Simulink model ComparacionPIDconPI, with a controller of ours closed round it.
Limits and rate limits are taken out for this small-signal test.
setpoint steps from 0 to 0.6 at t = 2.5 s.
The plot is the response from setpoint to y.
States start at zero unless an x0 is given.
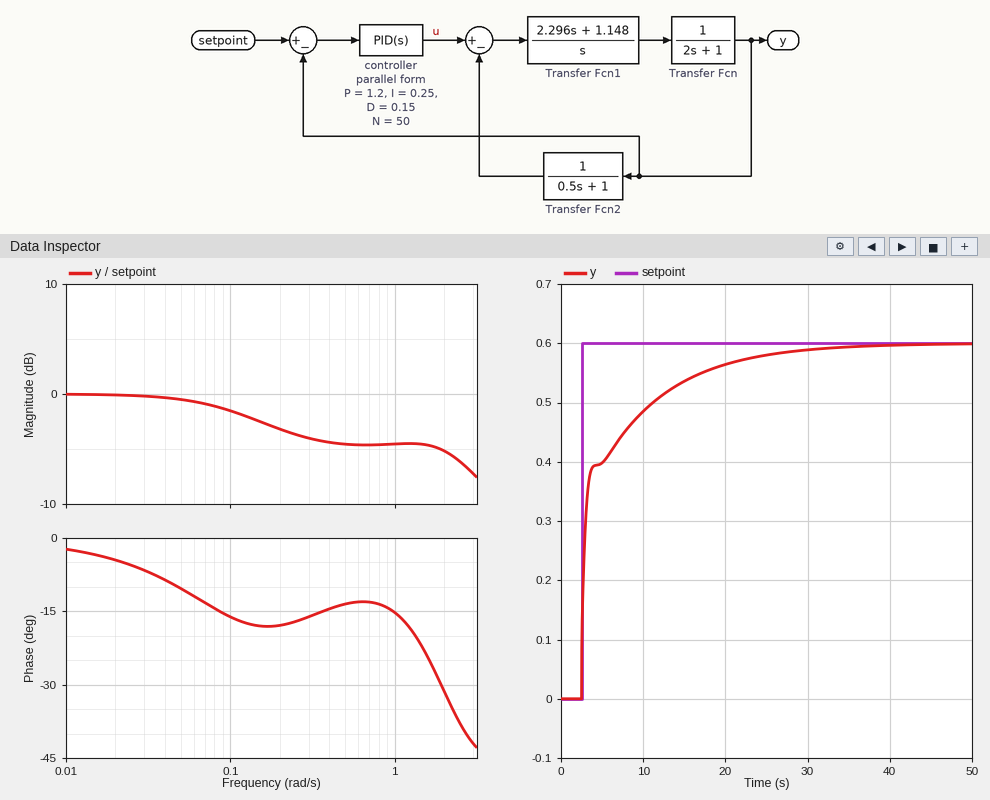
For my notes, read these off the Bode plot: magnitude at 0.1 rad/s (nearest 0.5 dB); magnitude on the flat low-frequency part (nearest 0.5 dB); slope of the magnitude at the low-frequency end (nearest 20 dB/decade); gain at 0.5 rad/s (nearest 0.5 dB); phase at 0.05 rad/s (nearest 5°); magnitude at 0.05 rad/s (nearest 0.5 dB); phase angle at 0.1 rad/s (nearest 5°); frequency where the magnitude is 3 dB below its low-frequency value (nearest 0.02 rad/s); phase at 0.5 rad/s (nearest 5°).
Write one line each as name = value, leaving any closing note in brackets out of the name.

magnitude at 0.1 rad/s = -1.5 dB
magnitude on the flat low-frequency part = 0.0 dB
slope of the magnitude at the low-frequency end = 0 dB/decade
gain at 0.5 rad/s = -4.5 dB
phase at 0.05 rad/s = -10°
magnitude at 0.05 rad/s = -0.5 dB
phase angle at 0.1 rad/s = -15°
frequency where the magnitude is 3 dB below its low-frequency value = 0.18 rad/s
phase at 0.5 rad/s = -15°
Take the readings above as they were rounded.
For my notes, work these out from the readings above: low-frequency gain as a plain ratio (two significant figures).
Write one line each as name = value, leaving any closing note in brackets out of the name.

low-frequency gain as a plain ratio = 1.0
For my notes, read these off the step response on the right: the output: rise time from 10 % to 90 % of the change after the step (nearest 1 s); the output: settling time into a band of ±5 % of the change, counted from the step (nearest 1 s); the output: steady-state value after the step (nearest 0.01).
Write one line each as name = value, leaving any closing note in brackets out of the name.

the output: rise time from 10 % to 90 % of the change after the step = 13 s
the output: settling time into a band of ±5 % of the change, counted from the step = 19 s
the output: steady-state value after the step = 0.60
